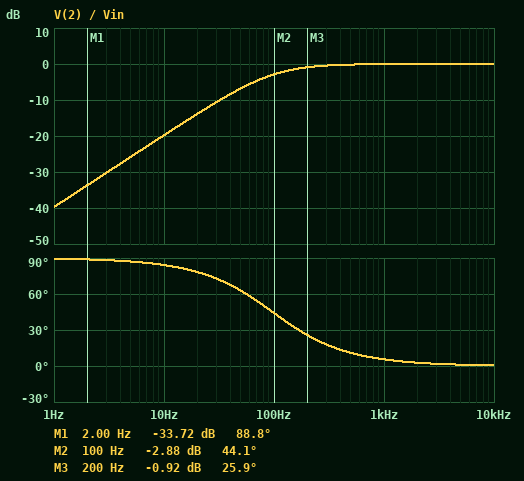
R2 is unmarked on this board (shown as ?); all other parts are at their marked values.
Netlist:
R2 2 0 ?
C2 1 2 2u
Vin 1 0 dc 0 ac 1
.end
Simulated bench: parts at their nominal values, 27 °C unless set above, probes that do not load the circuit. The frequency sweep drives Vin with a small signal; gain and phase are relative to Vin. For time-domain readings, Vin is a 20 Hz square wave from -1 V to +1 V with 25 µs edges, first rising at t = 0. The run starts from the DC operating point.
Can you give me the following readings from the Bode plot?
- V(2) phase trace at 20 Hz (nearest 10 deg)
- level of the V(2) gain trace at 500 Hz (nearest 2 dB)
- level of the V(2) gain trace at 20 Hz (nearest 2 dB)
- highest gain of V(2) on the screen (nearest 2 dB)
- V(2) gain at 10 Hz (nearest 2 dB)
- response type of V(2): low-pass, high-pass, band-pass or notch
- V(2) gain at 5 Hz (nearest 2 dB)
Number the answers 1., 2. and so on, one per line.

1. 80 deg
2. 0 dB
3. -14 dB
4. 0 dB
5. -20 dB
6. high-pass
7. -26 dB
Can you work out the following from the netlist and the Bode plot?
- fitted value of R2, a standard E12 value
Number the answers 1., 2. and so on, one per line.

1. 820 Ω
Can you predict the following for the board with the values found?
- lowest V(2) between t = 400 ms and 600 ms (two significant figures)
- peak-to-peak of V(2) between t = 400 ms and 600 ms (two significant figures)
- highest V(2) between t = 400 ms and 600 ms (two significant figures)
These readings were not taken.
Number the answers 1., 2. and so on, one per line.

1. -2.0 V
2. 4.0 V
3. 2.0 V
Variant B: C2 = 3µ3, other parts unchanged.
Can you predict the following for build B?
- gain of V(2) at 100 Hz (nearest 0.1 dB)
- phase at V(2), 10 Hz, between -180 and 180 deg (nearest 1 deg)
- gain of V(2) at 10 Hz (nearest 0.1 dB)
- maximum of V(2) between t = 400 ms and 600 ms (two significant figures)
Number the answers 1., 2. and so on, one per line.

1. -1.3 dB
2. 80 deg
3. -15.5 dB
4. 2.0 V
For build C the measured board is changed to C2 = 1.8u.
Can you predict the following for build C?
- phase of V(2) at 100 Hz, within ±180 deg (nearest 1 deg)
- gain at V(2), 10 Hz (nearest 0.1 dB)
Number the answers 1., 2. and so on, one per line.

1. 47 deg
2. -20.7 dB
